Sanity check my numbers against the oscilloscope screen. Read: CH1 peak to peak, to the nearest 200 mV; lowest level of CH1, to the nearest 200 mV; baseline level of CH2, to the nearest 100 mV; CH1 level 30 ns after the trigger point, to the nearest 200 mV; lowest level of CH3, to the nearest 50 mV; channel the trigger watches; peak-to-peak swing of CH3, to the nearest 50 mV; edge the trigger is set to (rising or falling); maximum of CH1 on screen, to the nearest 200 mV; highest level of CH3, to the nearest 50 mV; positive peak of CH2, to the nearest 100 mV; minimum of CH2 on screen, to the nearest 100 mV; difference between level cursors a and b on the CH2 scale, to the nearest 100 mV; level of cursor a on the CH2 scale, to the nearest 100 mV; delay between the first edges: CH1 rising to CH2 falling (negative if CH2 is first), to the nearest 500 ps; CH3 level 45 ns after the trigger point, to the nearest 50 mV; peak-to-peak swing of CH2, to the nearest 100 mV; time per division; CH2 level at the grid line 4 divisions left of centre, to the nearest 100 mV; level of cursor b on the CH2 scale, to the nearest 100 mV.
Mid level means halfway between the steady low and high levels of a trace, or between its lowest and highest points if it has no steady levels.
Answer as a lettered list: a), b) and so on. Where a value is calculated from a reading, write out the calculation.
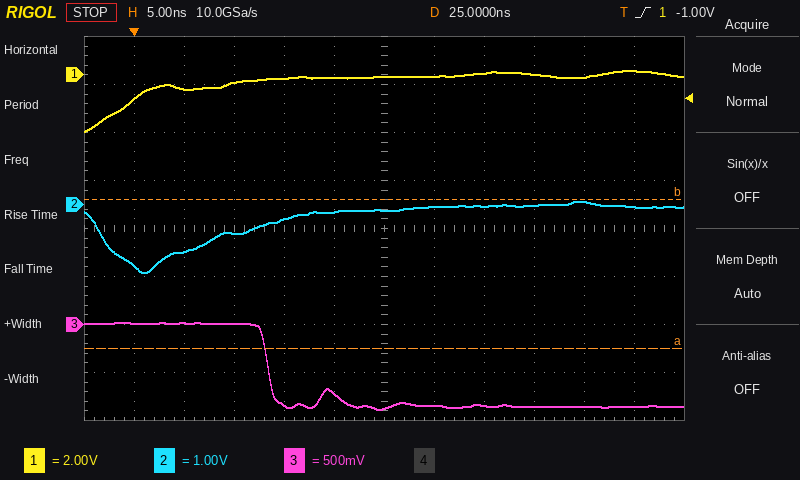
a) 200 mV − (-2.4 V) = 2.6 V
b) -2.4 V
c) -100 mV
d) 0.0 V
e) -900 mV
f) CH1
g) 0 mV − (-900 mV) = 900 mV
h) rising
i) 200 mV
j) 0 mV
k) 100 mV
l) -1.4 V
m) 3.1 V
n) -3.0 V
o) -3.0 ns
p) -850 mV
q) 100 mV − (-1.4 V) = 1.5 V
r) 5 ns
s) -1.0 V
t) 100 mV
